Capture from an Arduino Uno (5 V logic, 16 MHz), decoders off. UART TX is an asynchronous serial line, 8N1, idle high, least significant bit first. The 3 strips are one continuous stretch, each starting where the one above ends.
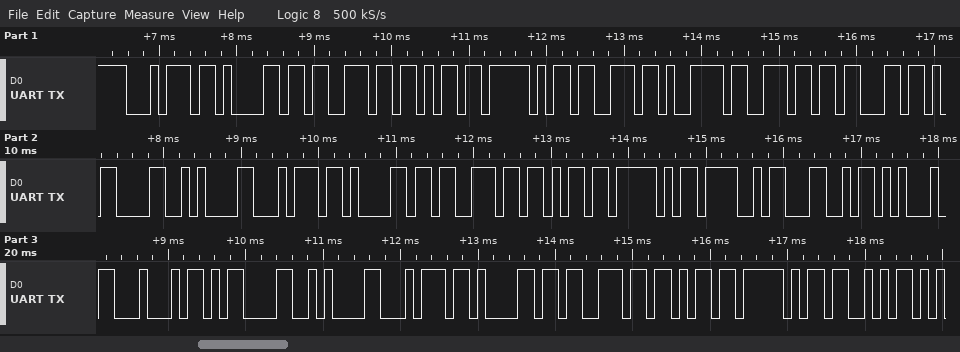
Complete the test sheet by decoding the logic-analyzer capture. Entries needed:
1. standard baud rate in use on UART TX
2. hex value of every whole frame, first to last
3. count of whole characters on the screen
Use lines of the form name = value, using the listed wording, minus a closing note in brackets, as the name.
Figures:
standard baud rate in use on UART TX = 9600 baud
hex value of every whole frame, first to last = 74 61 73 6B 5F 73 79 6E 63 0D 0A 74 61 73 6B 5F 4F 4C 45 44 0D 0A 74 61 73 6B 5F 53
count of whole characters on the screen = 28
